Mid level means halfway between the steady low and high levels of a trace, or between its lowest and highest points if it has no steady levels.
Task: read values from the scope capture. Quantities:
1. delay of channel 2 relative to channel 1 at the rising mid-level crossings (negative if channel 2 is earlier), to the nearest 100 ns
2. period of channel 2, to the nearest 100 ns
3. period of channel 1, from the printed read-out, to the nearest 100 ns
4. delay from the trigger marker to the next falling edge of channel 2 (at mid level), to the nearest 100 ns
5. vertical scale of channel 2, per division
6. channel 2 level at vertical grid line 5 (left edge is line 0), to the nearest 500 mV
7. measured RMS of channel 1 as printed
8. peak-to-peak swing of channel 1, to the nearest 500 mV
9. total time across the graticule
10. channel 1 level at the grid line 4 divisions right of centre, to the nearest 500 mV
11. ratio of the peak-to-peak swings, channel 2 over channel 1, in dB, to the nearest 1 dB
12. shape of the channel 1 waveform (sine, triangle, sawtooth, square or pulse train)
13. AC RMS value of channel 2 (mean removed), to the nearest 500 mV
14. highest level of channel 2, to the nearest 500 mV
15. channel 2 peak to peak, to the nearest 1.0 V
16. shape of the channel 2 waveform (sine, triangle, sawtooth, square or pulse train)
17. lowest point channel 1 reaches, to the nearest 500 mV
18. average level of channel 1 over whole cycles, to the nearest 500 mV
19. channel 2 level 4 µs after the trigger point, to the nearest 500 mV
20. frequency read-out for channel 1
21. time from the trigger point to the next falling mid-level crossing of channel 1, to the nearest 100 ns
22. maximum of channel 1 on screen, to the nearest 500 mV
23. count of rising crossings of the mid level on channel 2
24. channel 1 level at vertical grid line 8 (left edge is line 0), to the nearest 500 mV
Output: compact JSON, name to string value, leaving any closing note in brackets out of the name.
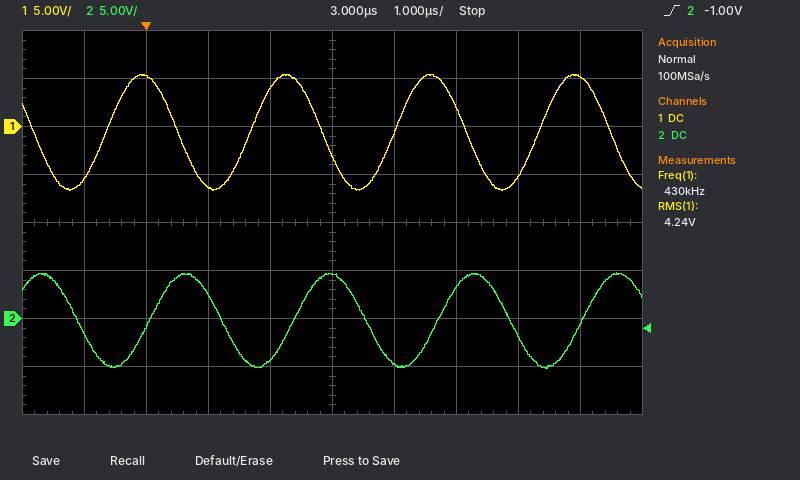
{"delay of channel 2 relative to channel 1 at the rising mid-level crossings (negative if channel 2 is earlier), to the nearest 100 ns": "+700 ns", "period of channel 2, to the nearest 100 ns": "2.3 µs", "period of channel 1, from the printed read-out, to the nearest 100 ns": "2.3 µs", "delay from the trigger marker to the next falling edge of channel 2 (at mid level), to the nearest 100 ns": "1.2 µs", "vertical scale of channel 2, per division": "5 V", "channel 2 level at vertical grid line 5 (left edge is line 0), to the nearest 500 mV": "4.5 V", "measured RMS of channel 1 as printed": "4.24 V", "peak-to-peak swing of channel 1, to the nearest 500 mV": "12.0 V", "total time across the graticule": "10 µs", "channel 1 level at the grid line 4 divisions right of centre, to the nearest 500 mV": "5.0 V", "ratio of the peak-to-peak swings, channel 2 over channel 1, in dB, to the nearest 1 dB": "-2 dB", "shape of the channel 1 waveform": "sine", "AC RMS value of channel 2 (mean removed), to the nearest 500 mV": "3.5 V", "highest level of channel 2, to the nearest 500 mV": "5.0 V", "channel 2 peak to peak, to the nearest 1.0 V": "10.0 V", "shape of the channel 2 waveform": "sine", "lowest point channel 1 reaches, to the nearest 500 mV": "-6.5 V", "average level of channel 1 over whole cycles, to the nearest 500 mV": "-500 mV", "channel 2 level 4 µs after the trigger point, to the nearest 500 mV": "-4.5 V", "frequency read-out for channel 1": "430 kHz", "time from the trigger point to the next falling mid-level crossing of channel 1, to the nearest 100 ns": "500 ns", "maximum of channel 1 on screen, to the nearest 500 mV": "5.5 V", "count of rising crossings of the mid level on channel 2": "4", "channel 1 level at vertical grid line 8 (left edge is line 0), to the nearest 500 mV": "-5.0 V"}
